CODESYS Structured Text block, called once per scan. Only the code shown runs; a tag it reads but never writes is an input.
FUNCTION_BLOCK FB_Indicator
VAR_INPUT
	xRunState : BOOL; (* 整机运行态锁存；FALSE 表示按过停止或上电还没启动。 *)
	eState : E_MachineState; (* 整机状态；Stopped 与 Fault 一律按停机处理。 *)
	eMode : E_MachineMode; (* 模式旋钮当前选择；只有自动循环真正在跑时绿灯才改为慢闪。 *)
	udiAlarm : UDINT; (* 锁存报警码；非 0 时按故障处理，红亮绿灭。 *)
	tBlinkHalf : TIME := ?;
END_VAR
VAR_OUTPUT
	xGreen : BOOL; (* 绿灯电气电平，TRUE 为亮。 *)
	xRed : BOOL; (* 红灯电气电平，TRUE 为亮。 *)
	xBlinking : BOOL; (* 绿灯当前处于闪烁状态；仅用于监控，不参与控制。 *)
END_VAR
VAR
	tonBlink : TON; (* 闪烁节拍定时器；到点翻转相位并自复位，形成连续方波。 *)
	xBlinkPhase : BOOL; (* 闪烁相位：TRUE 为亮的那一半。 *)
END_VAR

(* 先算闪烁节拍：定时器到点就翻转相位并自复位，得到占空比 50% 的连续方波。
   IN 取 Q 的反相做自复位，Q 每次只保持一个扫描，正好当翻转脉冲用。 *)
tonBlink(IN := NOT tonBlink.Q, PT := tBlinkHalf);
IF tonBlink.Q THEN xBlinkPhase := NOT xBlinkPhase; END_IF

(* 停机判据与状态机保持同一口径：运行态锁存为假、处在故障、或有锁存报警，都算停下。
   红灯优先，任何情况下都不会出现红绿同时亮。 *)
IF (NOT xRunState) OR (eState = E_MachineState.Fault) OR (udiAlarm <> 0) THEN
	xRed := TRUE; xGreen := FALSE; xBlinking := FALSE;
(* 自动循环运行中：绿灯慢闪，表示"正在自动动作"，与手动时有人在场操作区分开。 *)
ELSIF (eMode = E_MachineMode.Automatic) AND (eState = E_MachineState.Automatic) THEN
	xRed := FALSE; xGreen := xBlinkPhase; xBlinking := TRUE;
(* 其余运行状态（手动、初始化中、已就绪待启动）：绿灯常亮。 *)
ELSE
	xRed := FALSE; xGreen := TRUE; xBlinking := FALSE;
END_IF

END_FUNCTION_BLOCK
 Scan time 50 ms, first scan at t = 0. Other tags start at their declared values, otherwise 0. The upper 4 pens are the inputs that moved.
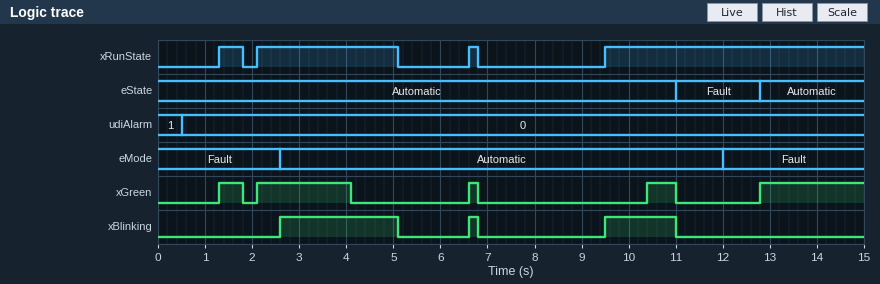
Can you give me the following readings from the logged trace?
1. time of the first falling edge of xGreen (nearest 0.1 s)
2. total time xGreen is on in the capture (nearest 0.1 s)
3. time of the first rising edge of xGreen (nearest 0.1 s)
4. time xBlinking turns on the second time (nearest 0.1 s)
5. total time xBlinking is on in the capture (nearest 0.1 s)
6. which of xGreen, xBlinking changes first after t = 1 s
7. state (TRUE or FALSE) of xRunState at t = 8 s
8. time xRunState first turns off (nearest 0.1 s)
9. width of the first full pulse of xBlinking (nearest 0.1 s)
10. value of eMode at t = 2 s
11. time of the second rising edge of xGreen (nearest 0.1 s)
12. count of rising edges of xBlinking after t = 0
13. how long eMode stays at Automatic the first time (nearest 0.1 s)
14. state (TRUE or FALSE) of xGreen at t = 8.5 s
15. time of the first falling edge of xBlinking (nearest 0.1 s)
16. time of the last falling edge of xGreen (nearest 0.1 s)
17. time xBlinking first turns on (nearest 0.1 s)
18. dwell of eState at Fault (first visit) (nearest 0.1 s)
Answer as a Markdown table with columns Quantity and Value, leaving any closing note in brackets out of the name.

| Quantity | Value |
|---|---|
| time of the first falling edge of xGreen | 1.8 s |
| total time xGreen is on in the capture | 5.5 s |
| time of the first rising edge of xGreen | 1.3 s |
| time xBlinking turns on the second time | 6.6 s |
| total time xBlinking is on in the capture | 4.2 s |
| which of xGreen, xBlinking changes first after t = 1 s | xGreen |
| state (TRUE or FALSE) of xRunState at t = 8 s | FALSE |
| time xRunState first turns off | 1.8 s |
| width of the first full pulse of xBlinking | 2.5 s |
| value of eMode at t = 2 s | Fault |
| time of the second rising edge of xGreen | 2.1 s |
| count of rising edges of xBlinking after t = 0 | 3 |
| how long eMode stays at Automatic the first time | 9.4 s |
| state (TRUE or FALSE) of xGreen at t = 8.5 s | FALSE |
| time of the first falling edge of xBlinking | 5.1 s |
| time of the last falling edge of xGreen | 11.0 s |
| time xBlinking first turns on | 2.6 s |
| dwell of eState at Fault (first visit) | 1.8 s |
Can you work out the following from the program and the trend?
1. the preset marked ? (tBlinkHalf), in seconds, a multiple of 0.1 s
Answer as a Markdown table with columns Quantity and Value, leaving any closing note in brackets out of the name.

| Quantity | Value |
|---|---|
| the preset marked ? (tBlinkHalf), in seconds, a multiple of 0.1 s | 2.0 s |
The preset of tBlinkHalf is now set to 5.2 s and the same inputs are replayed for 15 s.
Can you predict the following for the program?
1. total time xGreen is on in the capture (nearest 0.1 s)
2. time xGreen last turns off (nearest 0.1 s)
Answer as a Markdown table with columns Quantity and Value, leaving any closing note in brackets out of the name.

| Quantity | Value |
|---|---|
| total time xGreen is on in the capture | 4.4 s |
| time xGreen last turns off | 10.5 s |
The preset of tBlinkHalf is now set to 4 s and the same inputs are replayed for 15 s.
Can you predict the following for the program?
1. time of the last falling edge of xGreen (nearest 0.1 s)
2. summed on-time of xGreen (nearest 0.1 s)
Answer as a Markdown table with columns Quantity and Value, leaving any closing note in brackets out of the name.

| Quantity | Value |
|---|---|
| time of the last falling edge of xGreen | 6.8 s |
| summed on-time of xGreen | 4.5 s |
